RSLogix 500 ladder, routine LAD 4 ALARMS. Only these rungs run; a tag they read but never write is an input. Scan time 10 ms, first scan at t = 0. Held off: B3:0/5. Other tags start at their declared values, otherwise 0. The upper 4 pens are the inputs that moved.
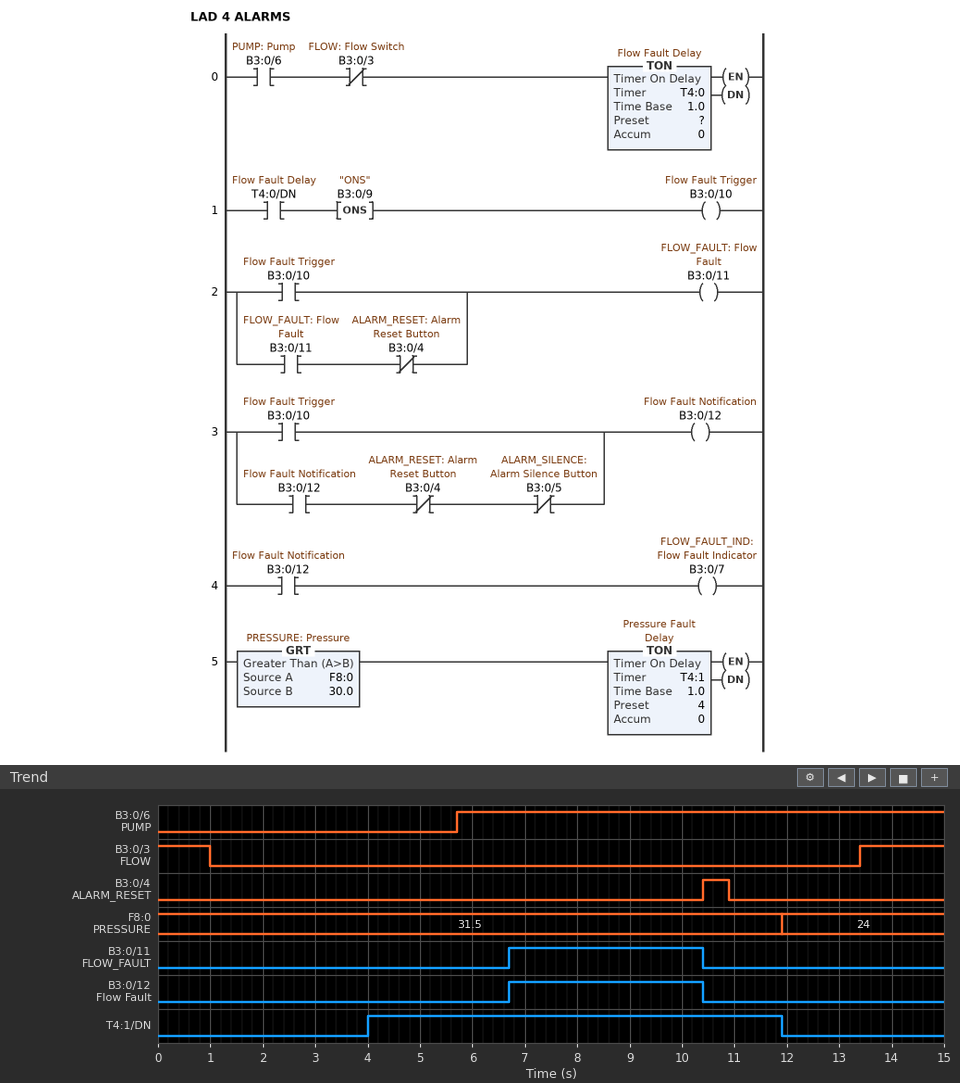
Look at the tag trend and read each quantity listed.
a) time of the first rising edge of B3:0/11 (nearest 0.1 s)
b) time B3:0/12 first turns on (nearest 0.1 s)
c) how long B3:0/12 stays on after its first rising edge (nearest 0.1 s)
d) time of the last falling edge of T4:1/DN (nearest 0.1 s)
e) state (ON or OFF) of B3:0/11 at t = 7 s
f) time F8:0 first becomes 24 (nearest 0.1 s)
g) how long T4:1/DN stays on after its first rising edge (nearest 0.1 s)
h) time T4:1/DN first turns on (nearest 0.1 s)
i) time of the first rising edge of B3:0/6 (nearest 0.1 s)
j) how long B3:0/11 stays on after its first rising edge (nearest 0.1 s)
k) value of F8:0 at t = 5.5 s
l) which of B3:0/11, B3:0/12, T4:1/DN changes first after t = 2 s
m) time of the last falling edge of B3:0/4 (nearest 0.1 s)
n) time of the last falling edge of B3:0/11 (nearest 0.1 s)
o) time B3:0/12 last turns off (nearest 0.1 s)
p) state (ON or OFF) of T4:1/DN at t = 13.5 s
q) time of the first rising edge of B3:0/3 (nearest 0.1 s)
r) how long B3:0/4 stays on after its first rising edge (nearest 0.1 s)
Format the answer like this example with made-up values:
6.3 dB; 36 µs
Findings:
6.7 s; 6.7 s; 3.7 s; 11.9 s; ON; 11.9 s; 7.9 s; 4.0 s; 5.7 s; 3.7 s; 31.5; T4:1/DN; 10.9 s; 10.4 s; 10.4 s; OFF; 13.4 s; 0.5 s
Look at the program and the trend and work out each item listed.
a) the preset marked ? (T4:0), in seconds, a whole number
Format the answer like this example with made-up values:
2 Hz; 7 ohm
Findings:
1 s
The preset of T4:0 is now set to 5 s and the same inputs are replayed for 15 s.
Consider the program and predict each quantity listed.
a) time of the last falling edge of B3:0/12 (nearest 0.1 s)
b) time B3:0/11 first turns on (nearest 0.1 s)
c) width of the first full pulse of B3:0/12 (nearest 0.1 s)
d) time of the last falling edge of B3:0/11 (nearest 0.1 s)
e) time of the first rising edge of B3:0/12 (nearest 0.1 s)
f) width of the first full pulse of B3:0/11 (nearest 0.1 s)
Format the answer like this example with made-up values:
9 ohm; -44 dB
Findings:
10.7 s; 10.7 s; 0.0 s; 10.7 s; 10.7 s; 0.0 s
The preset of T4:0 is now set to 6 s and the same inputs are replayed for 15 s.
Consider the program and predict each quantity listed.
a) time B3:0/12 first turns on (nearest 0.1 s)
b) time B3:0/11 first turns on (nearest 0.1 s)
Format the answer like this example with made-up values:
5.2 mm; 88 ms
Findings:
11.7 s; 11.7 s
